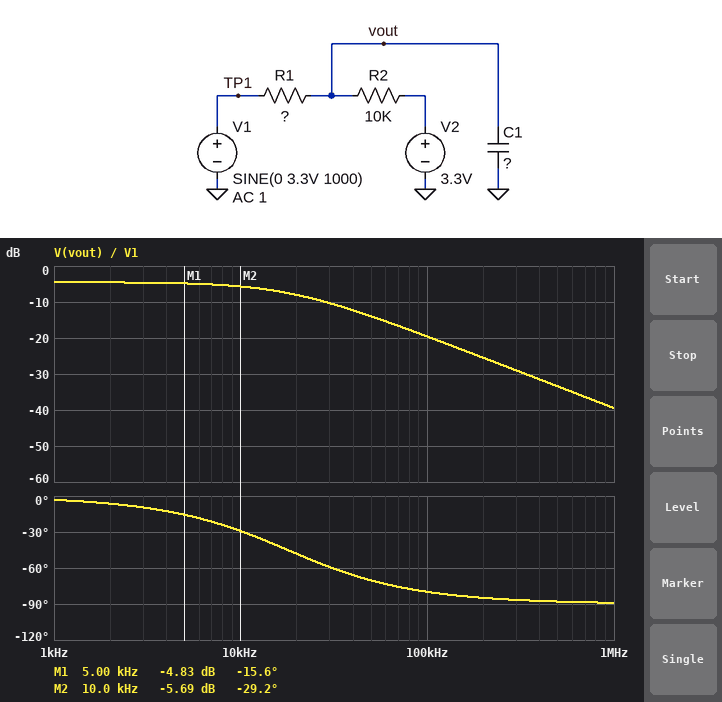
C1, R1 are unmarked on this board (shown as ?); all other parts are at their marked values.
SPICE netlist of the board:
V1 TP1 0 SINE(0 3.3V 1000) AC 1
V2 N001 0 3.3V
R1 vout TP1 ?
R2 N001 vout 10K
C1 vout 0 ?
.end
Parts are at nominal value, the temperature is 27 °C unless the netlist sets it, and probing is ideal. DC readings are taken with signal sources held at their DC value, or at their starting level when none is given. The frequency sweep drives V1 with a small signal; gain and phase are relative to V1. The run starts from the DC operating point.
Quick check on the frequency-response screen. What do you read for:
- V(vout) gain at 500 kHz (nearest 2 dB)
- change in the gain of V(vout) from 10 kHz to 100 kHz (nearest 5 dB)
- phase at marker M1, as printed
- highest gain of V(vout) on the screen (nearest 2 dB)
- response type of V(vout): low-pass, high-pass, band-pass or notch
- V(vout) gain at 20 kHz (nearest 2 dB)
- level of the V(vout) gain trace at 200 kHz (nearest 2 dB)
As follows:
-34 dB
-15 dB
-15.6 deg
-4 dB
low-pass
-8 dB
-26 dB
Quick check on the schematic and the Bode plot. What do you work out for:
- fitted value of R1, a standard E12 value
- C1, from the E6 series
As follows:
6.8 kΩ
2.2 nF
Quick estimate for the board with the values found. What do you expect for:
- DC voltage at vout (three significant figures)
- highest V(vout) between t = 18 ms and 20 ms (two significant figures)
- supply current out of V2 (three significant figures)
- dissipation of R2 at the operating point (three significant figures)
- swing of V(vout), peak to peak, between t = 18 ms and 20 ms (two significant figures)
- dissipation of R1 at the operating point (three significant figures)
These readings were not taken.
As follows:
1.34 V
3.3 V
196 µA
386 µW
3.9 V
262 µW
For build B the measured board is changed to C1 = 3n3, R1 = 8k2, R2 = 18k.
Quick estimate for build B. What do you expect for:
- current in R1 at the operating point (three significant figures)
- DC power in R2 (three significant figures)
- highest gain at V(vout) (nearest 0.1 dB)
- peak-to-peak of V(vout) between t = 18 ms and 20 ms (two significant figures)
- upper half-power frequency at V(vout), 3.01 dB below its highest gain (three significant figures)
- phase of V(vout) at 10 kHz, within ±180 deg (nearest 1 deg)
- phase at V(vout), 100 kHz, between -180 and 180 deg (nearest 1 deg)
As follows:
126 µA
286 µW
-3.3 dB
4.5 V
8.56 kHz
-49 deg
-85 deg
